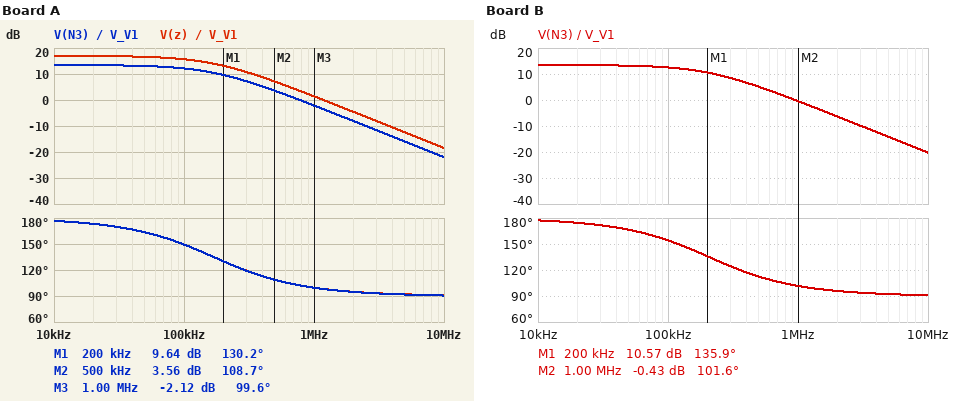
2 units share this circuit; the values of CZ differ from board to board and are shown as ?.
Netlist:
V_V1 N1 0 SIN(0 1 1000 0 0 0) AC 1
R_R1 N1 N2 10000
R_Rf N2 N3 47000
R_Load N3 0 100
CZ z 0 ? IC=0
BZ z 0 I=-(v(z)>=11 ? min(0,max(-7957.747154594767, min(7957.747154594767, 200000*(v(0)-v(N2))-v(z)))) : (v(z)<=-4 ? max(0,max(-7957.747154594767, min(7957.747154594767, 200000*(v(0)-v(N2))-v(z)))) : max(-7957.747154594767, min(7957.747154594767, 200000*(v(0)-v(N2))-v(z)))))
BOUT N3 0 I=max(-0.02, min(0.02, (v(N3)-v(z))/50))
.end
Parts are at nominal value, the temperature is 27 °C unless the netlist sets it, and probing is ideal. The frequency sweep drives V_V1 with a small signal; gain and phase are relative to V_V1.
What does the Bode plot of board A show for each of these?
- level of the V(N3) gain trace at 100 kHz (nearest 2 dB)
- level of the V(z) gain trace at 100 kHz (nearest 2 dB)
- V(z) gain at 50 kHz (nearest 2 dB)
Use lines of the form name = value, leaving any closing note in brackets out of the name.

level of the V(N3) gain trace at 100 kHz = 12 dB
level of the V(z) gain trace at 100 kHz = 16 dB
V(z) gain at 50 kHz = 16 dB
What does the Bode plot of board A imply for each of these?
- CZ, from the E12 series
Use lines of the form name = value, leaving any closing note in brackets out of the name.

CZ, from the E12 series = 22 mF
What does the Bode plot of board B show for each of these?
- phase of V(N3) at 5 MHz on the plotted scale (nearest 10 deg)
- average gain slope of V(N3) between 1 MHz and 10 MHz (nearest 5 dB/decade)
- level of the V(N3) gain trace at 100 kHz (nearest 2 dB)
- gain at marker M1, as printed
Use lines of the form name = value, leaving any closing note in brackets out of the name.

phase of V(N3) at 5 MHz on the plotted scale = 90 deg
average gain slope of V(N3) between 1 MHz and 10 MHz = -20 dB/decade
level of the V(N3) gain trace at 100 kHz = 12 dB
gain at marker M1, as printed = 10.57 dB
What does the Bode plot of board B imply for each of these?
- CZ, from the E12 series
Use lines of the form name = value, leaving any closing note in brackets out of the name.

CZ, from the E12 series = 18 mF
